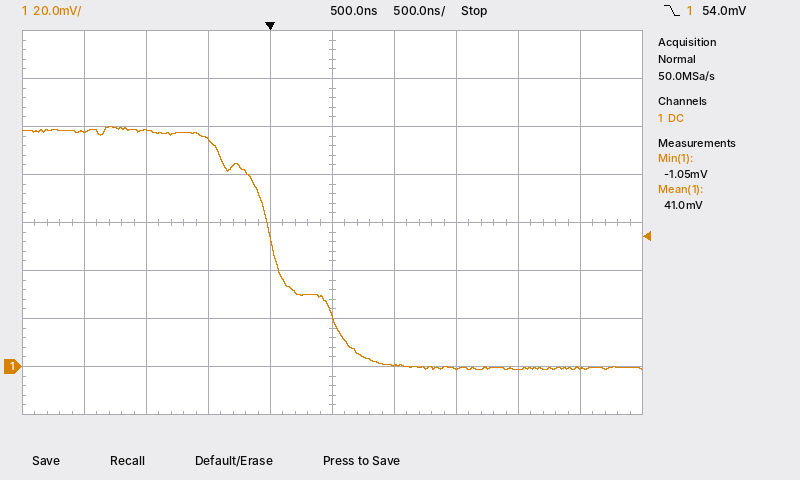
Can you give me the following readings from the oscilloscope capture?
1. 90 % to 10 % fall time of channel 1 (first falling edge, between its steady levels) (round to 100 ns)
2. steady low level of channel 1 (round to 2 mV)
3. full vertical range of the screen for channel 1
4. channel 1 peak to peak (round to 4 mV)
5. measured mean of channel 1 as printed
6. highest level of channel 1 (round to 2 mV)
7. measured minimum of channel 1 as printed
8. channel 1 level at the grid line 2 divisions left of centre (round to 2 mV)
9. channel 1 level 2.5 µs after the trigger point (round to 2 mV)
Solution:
1.0 µs
0 mV
160 mV
100 mV
41.0 mV
100 mV
-1.05 mV
94 mV
0 mV
